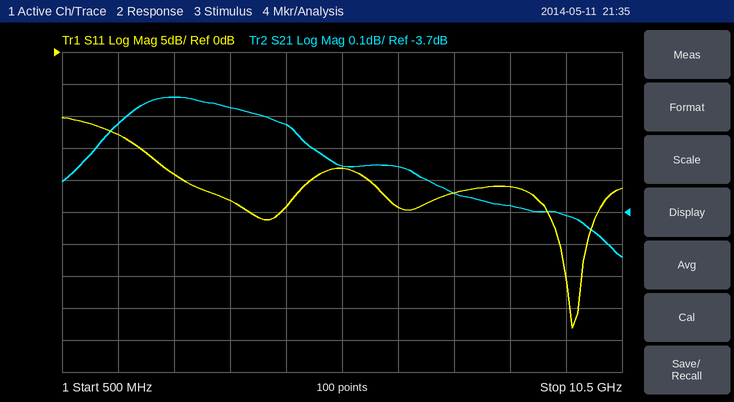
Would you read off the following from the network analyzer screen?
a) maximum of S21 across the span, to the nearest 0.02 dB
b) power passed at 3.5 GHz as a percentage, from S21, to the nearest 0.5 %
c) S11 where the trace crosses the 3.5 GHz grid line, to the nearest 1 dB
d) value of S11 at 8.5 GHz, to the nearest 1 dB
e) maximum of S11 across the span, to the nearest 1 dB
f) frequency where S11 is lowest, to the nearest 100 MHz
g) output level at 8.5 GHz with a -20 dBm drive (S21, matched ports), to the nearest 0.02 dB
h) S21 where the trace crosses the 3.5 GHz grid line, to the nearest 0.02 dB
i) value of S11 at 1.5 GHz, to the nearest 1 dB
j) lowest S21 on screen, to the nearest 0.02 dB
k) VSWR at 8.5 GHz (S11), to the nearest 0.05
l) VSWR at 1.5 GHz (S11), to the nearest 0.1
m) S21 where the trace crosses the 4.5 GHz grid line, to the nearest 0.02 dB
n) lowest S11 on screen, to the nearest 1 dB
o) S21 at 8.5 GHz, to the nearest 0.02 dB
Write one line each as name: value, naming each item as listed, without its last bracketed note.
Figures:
maximum of S21 across the span, to the nearest 0.02 dB: -3.34 dB
power passed at 3.5 GHz as a percentage, from S21, to the nearest 0.5 %: 46.0 %
S11 where the trace crosses the 3.5 GHz grid line, to the nearest 1 dB: -23 dB
value of S11 at 8.5 GHz, to the nearest 1 dB: -21 dB
maximum of S11 across the span, to the nearest 1 dB: -10 dB
frequency where S11 is lowest, to the nearest 100 MHz: 9.6 GHz
output level at 8.5 GHz with a -20 dBm drive (S21, matched ports), to the nearest 0.02 dB: -23.68 dBm
S21 where the trace crosses the 3.5 GHz grid line, to the nearest 0.02 dB: -3.38 dB
value of S11 at 1.5 GHz, to the nearest 1 dB: -13 dB
lowest S21 on screen, to the nearest 0.02 dB: -3.84 dB
VSWR at 8.5 GHz (S11), to the nearest 0.05: 1.20
VSWR at 1.5 GHz (S11), to the nearest 0.1: 1.6
S21 where the trace crosses the 4.5 GHz grid line, to the nearest 0.02 dB: -3.42 dB
lowest S11 on screen, to the nearest 1 dB: -43 dB
S21 at 8.5 GHz, to the nearest 0.02 dB: -3.68 dB
